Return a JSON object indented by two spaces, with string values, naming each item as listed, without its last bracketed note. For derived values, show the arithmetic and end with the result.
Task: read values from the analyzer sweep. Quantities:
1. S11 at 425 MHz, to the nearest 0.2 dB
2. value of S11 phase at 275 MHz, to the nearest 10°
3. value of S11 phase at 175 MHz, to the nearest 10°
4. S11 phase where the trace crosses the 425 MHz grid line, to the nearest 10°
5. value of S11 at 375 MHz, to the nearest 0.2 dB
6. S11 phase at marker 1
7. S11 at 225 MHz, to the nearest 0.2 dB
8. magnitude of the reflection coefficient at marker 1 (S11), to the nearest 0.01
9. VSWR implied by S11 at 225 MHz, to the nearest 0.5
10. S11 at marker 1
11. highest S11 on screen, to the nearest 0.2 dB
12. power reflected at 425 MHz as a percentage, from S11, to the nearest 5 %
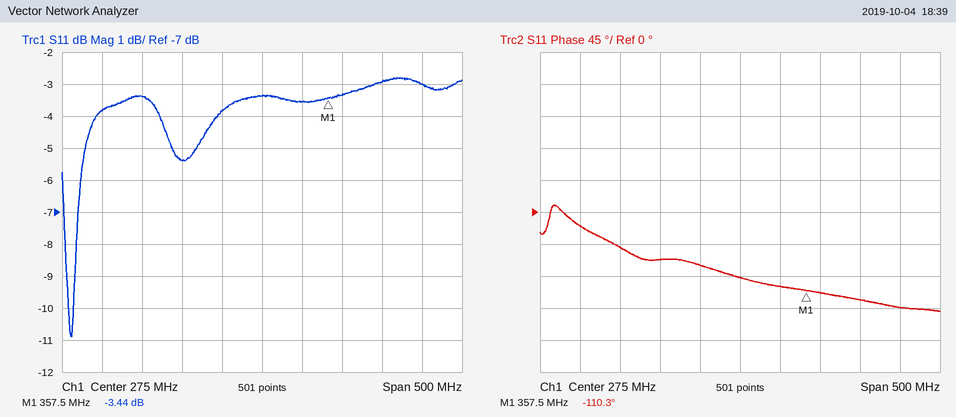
{
  "S11 at 425 MHz, to the nearest 0.2 dB": "-3.0 dB",
  "value of S11 phase at 275 MHz, to the nearest 10°": "-90°",
  "value of S11 phase at 175 MHz, to the nearest 10°": "-70°",
  "S11 phase where the trace crosses the 425 MHz grid line, to the nearest 10°": "-120°",
  "value of S11 at 375 MHz, to the nearest 0.2 dB": "-3.4 dB",
  "S11 phase at marker 1": "-110.3°",
  "S11 at 225 MHz, to the nearest 0.2 dB": "-3.8 dB",
  "magnitude of the reflection coefficient at marker 1 (S11), to the nearest 0.01": "10^(-3.44/20) ≈ 0.67",
  "VSWR implied by S11 at 225 MHz, to the nearest 0.5": "|Γ| = 10^(-3.8/20) = 0.6457; VSWR = (1 + 0.6457)/(1 − 0.6457) ≈ 4.64, so 4.5 to the nearest 0.5",
  "S11 at marker 1": "-3.44 dB",
  "highest S11 on screen, to the nearest 0.2 dB": "-2.8 dB",
  "power reflected at 425 MHz as a percentage, from S11, to the nearest 5 %": "10^(-3/10) ≈ 50 %"
}
